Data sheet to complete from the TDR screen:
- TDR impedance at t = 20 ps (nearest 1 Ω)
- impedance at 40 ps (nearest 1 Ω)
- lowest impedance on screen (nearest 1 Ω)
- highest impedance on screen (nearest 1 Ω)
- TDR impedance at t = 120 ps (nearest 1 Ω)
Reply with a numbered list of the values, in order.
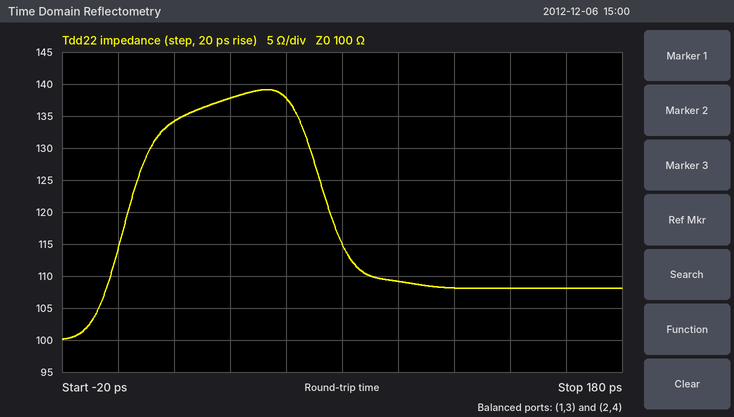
1. 134 Ω
2. 138 Ω
3. 100 Ω
4. 139 Ω
5. 108 Ω
